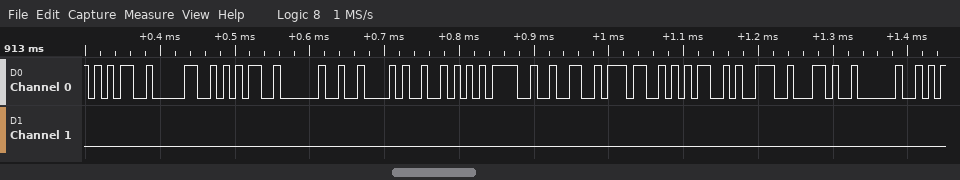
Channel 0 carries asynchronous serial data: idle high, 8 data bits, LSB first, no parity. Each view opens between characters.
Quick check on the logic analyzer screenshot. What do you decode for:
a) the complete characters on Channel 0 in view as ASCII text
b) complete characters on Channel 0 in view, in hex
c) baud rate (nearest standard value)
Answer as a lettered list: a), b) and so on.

a) "505 BR=2759, "
b) 35, 30, 35, 20, 42, 52, 3D, 32, 37, 35, 39, 2C, 20
c) 115200 baud
